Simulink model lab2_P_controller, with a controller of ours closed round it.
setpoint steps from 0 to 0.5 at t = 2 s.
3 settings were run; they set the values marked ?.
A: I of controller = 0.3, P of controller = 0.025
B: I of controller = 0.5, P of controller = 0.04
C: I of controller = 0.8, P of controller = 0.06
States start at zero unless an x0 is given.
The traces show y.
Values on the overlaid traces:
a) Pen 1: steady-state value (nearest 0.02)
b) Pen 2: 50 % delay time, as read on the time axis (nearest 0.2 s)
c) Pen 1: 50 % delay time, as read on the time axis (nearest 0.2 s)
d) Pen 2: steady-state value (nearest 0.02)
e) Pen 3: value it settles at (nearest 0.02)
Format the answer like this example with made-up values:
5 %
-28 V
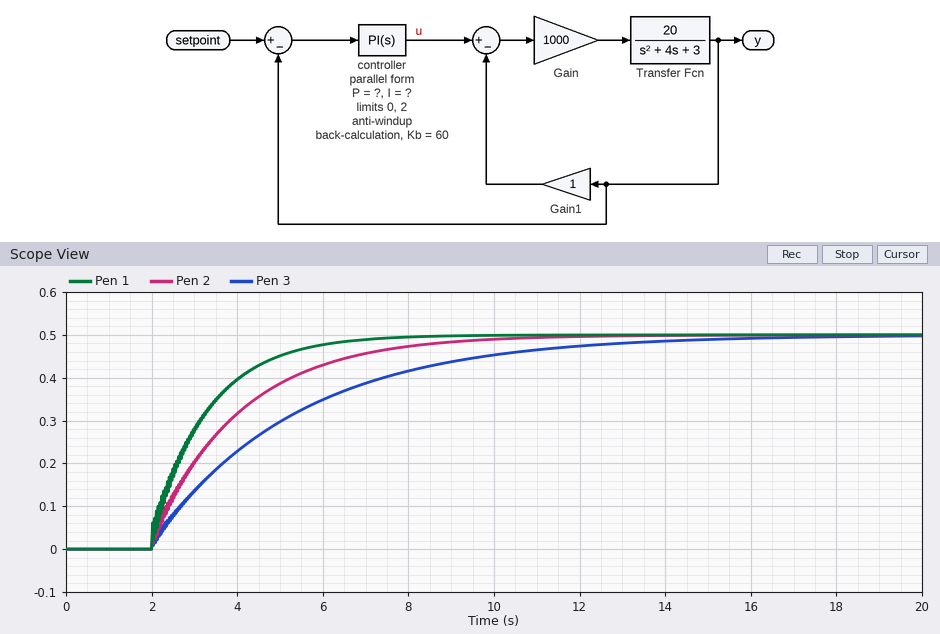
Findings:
0.50
3.4 s
2.8 s
0.50
0.50
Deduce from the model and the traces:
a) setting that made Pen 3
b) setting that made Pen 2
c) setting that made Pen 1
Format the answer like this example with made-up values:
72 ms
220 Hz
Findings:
A
B
C
